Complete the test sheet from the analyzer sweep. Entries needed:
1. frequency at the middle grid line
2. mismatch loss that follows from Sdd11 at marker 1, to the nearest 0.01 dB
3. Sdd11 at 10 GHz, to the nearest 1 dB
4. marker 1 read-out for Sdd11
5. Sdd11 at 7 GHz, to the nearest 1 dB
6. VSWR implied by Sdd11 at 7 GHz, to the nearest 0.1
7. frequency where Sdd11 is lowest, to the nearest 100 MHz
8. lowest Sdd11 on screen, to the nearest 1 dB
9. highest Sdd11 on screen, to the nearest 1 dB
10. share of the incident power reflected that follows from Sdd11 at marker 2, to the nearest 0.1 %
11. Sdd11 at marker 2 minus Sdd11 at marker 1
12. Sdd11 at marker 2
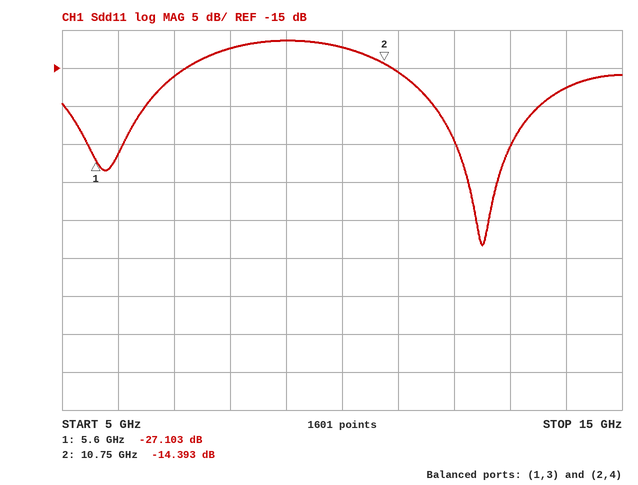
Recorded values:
10 GHz
0.01 dB
-12 dB
-27.103 dB
-16 dB
1.4
12.5 GHz
-38 dB
-11 dB
3.6 %
12.710 dB
-14.393 dB
